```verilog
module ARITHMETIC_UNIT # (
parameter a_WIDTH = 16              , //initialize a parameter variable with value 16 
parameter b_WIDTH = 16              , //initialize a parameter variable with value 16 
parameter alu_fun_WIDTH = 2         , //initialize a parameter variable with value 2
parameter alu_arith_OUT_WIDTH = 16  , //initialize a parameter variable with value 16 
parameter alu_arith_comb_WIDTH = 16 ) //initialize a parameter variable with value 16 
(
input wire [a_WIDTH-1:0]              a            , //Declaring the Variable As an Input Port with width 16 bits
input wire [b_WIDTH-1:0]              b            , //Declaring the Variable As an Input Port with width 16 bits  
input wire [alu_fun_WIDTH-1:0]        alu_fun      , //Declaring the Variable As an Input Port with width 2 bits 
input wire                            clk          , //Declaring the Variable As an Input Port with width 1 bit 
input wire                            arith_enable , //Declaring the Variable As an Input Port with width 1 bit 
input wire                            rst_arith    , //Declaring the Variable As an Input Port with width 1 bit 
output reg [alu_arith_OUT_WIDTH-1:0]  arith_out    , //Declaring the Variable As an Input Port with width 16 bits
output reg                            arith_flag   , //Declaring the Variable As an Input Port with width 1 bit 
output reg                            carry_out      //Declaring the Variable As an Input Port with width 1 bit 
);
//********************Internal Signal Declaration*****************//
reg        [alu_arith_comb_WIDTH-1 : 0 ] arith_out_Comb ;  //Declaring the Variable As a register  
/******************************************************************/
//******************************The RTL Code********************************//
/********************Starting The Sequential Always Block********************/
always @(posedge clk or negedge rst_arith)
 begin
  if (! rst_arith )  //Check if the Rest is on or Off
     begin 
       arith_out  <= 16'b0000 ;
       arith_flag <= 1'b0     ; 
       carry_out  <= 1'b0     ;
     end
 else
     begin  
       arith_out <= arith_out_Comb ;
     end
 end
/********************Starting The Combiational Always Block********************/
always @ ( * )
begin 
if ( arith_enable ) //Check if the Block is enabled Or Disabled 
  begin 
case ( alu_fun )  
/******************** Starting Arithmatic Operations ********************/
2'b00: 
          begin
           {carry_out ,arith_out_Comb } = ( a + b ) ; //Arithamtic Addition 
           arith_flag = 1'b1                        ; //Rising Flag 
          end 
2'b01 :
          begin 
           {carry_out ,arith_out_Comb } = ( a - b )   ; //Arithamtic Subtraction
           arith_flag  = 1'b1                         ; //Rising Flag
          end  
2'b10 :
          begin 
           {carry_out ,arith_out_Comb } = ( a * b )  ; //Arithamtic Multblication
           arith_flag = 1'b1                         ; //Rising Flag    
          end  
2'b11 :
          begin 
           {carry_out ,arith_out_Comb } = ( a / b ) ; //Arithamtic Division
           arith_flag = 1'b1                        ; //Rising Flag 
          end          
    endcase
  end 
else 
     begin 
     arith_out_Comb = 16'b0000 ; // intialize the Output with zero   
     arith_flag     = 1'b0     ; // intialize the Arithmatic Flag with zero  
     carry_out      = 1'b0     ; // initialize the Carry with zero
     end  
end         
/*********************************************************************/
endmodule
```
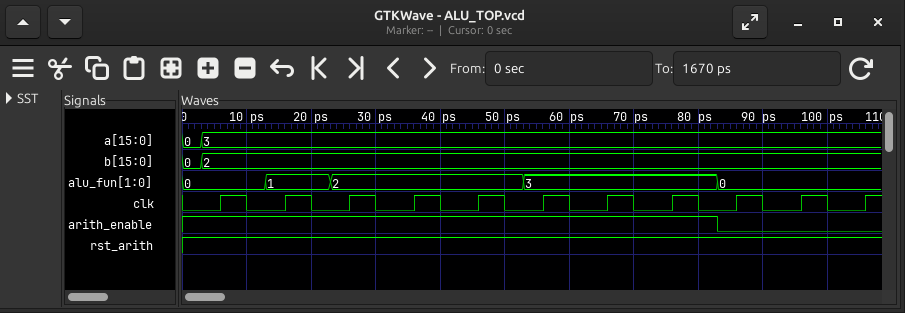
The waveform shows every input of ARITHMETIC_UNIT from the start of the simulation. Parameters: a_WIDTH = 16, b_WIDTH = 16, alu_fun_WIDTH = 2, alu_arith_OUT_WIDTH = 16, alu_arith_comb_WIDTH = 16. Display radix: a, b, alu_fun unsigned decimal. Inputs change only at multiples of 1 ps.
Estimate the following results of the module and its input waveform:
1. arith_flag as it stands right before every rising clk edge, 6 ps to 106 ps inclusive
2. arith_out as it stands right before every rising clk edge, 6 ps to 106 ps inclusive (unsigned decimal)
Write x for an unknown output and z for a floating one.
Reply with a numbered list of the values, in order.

1. 1 1 1 1 1 1 1 1 0 0 0
2. x, 5, 1, 6, 6, 6, 1, 1, 1, 0, 0
